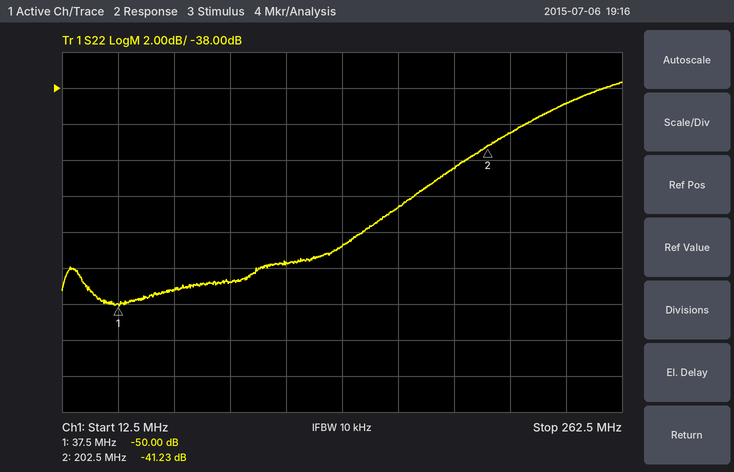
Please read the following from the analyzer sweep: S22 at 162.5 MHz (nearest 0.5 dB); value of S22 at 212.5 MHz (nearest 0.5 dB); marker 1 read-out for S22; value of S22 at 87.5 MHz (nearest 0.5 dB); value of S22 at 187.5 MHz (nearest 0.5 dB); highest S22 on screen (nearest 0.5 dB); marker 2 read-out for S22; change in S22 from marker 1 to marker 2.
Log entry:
-44.5 dB
-40.5 dB
-50.00 dB
-49.0 dB
-42.5 dB
-37.5 dB
-41.23 dB
8.77 dB
